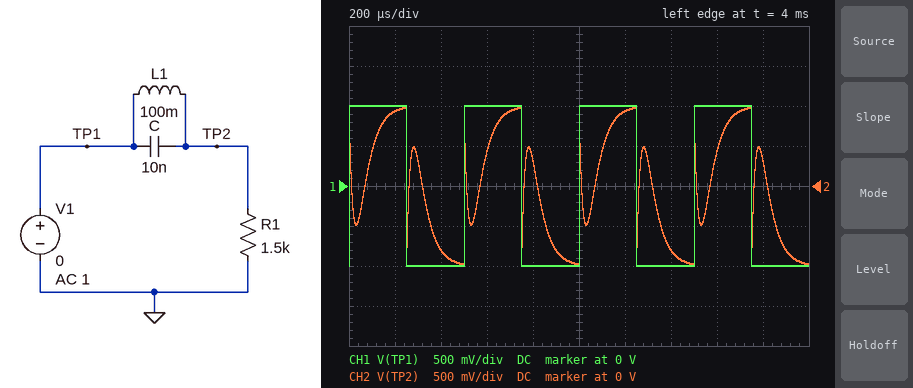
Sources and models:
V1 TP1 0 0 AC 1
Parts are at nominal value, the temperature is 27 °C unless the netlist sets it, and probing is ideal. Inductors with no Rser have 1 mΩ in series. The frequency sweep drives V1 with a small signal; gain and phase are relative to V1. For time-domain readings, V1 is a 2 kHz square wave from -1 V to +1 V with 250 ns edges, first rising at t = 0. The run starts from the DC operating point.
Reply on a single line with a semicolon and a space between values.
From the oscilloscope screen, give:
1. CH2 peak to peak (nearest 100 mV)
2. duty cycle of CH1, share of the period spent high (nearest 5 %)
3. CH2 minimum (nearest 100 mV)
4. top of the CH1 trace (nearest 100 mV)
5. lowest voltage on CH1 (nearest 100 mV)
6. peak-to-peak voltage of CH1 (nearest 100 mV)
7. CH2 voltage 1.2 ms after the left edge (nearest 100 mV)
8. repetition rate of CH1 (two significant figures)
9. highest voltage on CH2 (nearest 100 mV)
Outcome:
2.0 V; 50 %; -1.0 V; 1.0 V; -1.0 V; 2.0 V; 900 mV; 2.0 kHz; 1.0 V
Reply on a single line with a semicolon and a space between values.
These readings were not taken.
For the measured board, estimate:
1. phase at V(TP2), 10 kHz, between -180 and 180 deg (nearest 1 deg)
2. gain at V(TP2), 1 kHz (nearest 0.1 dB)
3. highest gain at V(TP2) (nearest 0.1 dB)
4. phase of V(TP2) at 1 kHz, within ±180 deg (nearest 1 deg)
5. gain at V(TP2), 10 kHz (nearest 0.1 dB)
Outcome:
55 deg; -0.8 dB; 0 dB; -24 deg; -4.8 dB
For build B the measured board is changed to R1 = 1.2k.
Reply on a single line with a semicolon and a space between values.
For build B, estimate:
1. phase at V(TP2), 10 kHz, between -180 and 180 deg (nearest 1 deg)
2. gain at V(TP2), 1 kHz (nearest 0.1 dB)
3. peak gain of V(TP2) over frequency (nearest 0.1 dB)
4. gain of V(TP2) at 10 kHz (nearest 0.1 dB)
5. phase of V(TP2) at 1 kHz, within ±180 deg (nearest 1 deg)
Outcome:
61 deg; -1.1 dB; 0 dB; -6.2 dB; -29 deg
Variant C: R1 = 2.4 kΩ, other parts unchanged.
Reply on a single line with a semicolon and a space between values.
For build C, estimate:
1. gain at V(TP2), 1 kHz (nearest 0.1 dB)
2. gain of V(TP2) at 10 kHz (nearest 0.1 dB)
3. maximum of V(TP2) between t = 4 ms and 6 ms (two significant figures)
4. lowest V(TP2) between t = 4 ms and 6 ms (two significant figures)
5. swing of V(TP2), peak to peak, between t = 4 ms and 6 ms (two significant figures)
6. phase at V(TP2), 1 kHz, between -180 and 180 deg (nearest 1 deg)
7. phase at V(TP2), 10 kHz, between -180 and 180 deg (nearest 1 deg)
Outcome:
-0.3 dB; -2.5 dB; 1.1 V; -1.1 V; 2.2 V; -15 deg; 42 deg
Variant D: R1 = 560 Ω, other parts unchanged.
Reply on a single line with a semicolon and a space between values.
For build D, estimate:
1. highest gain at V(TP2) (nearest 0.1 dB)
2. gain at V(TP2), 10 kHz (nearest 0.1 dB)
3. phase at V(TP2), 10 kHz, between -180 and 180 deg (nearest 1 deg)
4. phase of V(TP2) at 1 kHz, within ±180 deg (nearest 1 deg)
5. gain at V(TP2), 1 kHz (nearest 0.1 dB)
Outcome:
0 dB; -11.9 dB; 75 deg; -49 deg; -3.7 dB
